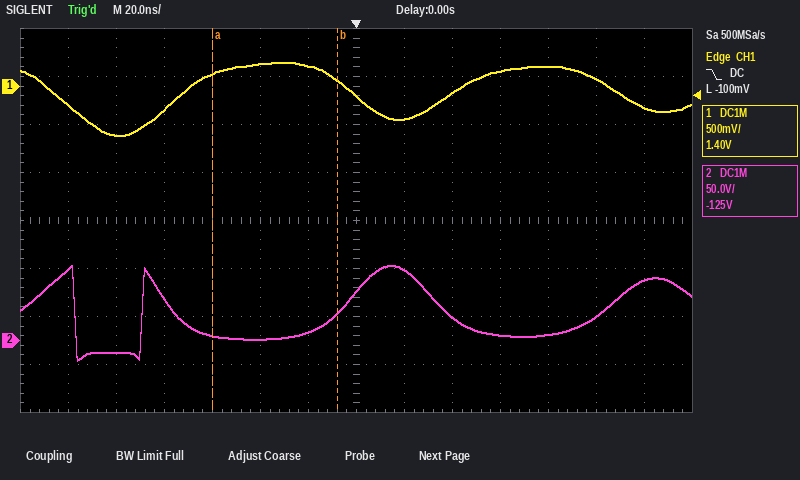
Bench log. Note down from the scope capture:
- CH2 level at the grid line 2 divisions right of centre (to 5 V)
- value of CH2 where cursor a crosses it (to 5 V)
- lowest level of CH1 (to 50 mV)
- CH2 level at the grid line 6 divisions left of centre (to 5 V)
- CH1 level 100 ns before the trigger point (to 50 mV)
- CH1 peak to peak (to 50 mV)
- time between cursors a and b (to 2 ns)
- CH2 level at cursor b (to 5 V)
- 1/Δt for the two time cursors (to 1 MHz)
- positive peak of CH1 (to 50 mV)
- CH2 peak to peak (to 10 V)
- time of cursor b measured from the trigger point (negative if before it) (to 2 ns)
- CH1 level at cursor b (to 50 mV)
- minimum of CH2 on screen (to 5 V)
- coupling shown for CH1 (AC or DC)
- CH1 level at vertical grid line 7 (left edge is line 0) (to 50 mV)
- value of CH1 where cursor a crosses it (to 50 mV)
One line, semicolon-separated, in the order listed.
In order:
25 V; 5 V; -500 mV; 75 V; -500 mV; 750 mV; 52 ns; 30 V; 19 MHz; 250 mV; 100 V; -8 ns; 50 mV; -20 V; DC; -100 mV; 150 mV
